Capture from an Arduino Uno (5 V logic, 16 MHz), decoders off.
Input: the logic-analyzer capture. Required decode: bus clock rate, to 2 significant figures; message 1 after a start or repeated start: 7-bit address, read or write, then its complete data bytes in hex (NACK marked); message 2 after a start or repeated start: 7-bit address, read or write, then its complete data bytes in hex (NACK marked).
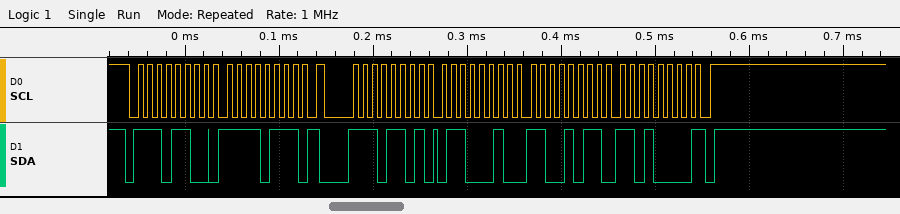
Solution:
100 kHz
0x76 write: F7
0x76 read: 62 CB D0 NACK
